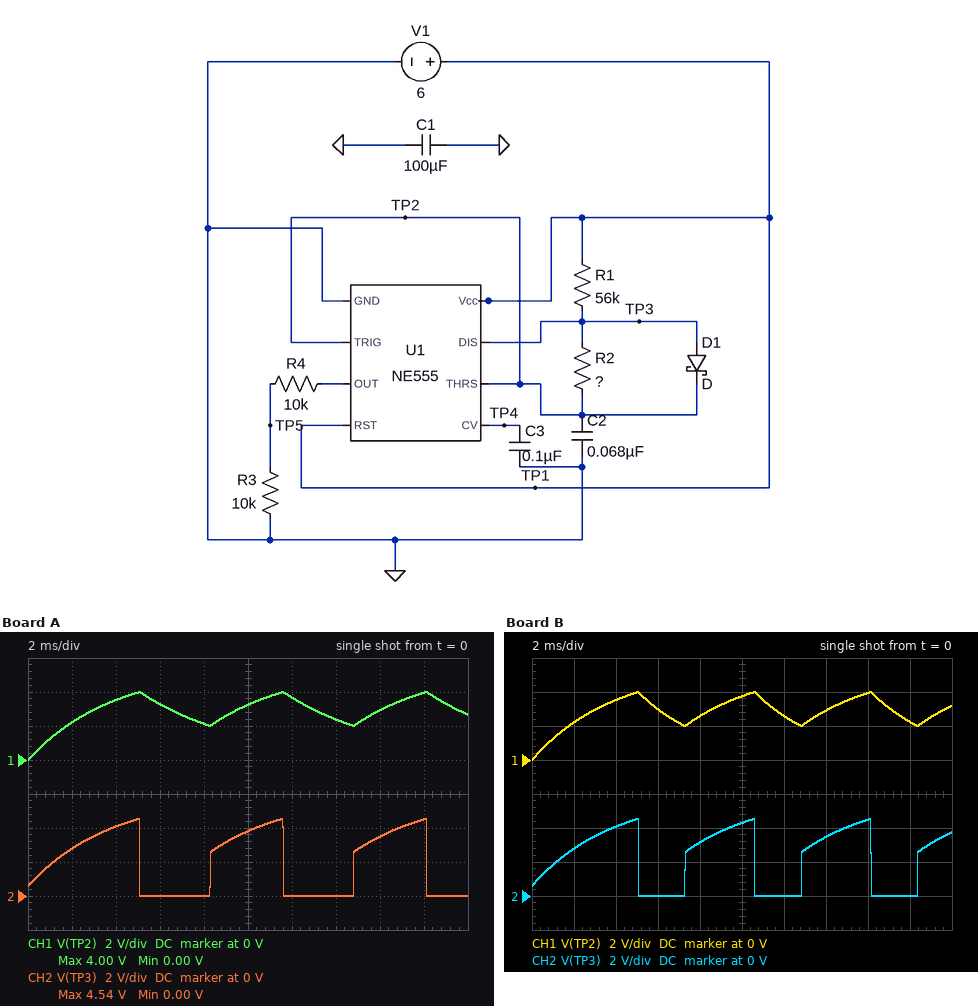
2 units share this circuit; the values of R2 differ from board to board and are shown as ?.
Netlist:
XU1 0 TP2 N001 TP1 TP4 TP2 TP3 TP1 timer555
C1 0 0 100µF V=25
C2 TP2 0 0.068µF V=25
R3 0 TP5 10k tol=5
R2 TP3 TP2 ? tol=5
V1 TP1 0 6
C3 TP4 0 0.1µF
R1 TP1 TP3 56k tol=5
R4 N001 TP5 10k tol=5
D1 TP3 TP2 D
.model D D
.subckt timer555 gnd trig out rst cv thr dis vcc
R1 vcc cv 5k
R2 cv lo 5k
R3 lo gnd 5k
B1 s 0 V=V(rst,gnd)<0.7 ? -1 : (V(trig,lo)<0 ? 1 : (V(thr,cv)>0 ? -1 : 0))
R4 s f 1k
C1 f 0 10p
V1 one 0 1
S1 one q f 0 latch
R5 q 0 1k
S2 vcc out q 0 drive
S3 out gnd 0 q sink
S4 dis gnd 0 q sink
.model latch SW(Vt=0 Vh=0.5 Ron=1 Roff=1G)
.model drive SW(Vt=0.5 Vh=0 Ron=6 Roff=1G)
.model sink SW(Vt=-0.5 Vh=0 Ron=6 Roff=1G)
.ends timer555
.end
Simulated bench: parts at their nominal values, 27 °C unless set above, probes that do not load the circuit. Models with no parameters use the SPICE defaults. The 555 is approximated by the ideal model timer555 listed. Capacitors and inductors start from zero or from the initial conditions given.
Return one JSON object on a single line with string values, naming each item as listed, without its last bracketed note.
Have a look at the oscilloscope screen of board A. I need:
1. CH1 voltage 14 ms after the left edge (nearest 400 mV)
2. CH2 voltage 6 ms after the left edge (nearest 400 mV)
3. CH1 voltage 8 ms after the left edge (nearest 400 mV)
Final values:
{"CH1 voltage 14 ms after the left edge": "2.4 V", "CH2 voltage 6 ms after the left edge": "0 V", "CH1 voltage 8 ms after the left edge": "2.0 V"}
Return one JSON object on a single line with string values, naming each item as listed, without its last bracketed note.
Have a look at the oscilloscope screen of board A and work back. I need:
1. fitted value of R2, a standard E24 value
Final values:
{"fitted value of R2, a standard E24 value": "68 kΩ"}
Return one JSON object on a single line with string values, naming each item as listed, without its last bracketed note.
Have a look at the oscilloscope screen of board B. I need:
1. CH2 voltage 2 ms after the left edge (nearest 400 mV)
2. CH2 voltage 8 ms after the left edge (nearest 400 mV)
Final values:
{"CH2 voltage 2 ms after the left edge": "2.8 V", "CH2 voltage 8 ms after the left edge": "3.2 V"}
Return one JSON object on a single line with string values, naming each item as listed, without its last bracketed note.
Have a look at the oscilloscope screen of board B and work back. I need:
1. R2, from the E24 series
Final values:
{"R2, from the E24 series": "47 kΩ"}
